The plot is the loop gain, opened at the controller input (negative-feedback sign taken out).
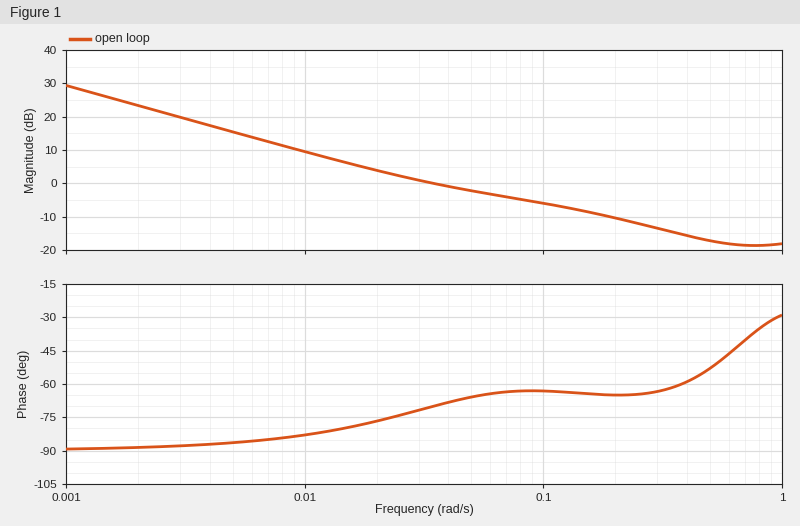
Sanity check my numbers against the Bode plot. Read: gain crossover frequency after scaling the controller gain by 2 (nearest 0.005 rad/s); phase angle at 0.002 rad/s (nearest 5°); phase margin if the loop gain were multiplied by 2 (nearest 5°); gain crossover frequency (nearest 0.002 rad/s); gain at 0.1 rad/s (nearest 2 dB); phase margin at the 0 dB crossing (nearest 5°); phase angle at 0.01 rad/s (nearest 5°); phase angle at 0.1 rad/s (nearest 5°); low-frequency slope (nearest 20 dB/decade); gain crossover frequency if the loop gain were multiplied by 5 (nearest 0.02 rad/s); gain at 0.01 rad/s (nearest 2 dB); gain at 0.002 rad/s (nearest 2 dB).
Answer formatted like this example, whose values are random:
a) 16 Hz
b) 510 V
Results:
a) 0.100 rad/s
b) -90°
c) 115°
d) 0.034 rad/s
e) -6 dB
f) 110°
g) -85°
h) -65°
i) -20 dB/decade
j) 0.32 rad/s
k) 10 dB
l) 24 dB
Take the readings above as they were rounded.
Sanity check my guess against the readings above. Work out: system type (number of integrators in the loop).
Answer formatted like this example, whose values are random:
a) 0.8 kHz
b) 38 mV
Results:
a) 1
